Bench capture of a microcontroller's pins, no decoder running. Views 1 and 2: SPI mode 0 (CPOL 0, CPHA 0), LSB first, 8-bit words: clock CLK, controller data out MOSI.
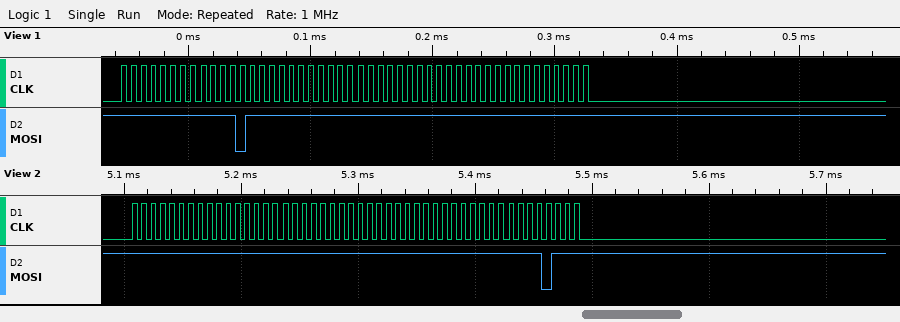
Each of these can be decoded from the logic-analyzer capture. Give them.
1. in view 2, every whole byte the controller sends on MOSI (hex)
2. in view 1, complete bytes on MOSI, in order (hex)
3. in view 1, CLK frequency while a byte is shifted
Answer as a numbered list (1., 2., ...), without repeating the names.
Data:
1. FF FF FF FF FF EF
2. FF EF FF FF FF FF
3. 125 kHz
